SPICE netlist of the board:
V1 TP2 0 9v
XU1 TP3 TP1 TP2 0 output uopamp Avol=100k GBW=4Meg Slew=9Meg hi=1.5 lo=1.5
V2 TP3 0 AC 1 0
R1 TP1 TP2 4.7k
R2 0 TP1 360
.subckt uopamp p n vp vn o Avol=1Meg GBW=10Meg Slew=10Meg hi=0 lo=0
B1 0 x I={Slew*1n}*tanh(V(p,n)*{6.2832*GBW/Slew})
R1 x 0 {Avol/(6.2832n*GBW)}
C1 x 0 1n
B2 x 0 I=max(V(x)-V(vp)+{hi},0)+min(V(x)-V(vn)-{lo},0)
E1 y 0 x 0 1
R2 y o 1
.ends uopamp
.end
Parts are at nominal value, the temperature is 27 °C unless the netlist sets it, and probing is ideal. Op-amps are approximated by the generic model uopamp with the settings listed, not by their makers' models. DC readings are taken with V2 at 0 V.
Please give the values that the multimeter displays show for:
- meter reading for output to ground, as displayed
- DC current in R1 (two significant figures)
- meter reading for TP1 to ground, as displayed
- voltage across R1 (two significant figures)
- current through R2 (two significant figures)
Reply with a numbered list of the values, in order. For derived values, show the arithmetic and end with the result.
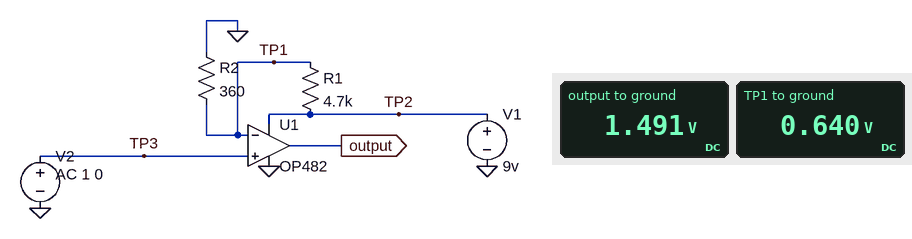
1. 1.491 V
2. (9 V - 640 mV) / 4.7 kΩ = 1.8 mA
3. 0.640 V
4. 9 V - 640 mV = 8.4 V
5. (640 mV) / 360 Ω = 1.8 mA
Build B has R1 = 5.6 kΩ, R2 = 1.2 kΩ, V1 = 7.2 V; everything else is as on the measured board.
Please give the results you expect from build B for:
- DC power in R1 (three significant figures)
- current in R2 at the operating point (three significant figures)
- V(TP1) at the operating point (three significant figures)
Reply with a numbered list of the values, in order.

1. 6.28 mW
2. 1.06 mA
3. 1.27 V
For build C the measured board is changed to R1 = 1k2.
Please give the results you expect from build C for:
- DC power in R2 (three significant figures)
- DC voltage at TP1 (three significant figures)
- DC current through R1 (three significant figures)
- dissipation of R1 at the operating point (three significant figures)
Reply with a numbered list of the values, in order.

1. 12.0 mW
2. 2.08 V
3. 5.77 mA
4. 39.9 mW
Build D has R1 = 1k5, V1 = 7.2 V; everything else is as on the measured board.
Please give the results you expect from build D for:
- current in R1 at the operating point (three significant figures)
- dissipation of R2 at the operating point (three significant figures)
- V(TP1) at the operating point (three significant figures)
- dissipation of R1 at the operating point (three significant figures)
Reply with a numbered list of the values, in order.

1. 3.87 mA
2. 5.39 mW
3. 1.39 V
4. 22.5 mW
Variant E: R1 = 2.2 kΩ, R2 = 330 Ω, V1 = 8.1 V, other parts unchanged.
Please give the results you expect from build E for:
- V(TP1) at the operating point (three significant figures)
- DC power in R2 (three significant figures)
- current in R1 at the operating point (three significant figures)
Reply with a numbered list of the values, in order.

1. 1.06 V
2. 3.38 mW
3. 3.20 mA
